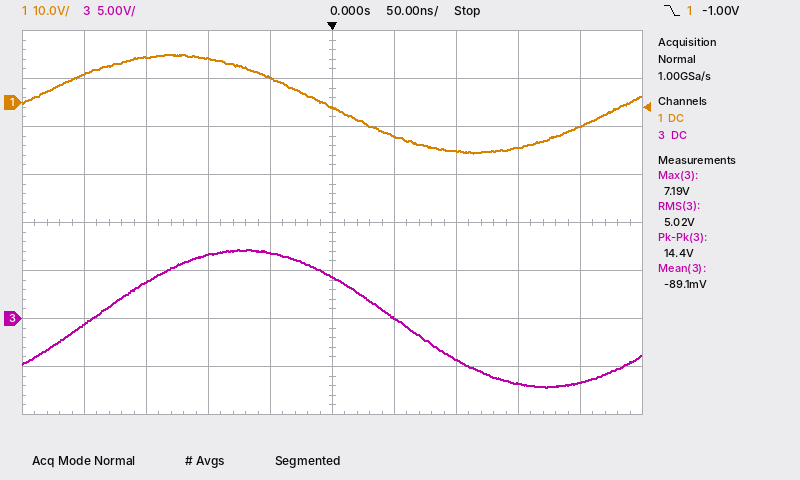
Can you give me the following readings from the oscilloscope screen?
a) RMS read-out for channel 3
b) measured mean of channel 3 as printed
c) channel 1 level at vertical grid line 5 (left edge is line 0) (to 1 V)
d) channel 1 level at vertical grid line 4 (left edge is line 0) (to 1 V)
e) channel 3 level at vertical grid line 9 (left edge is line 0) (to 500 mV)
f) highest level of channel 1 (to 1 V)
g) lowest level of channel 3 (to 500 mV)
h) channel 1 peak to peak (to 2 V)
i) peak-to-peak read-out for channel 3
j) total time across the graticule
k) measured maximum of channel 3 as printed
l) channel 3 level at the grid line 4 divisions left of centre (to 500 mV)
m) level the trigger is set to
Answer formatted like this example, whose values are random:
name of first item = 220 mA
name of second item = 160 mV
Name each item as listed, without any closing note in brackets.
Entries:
RMS read-out for channel 3 = 5.02 V
measured mean of channel 3 as printed = -89.1 mV
channel 1 level at vertical grid line 5 (left edge is line 0) = -1 V
channel 1 level at vertical grid line 4 (left edge is line 0) = 5 V
channel 3 level at vertical grid line 9 (left edge is line 0) = -6.5 V
highest level of channel 1 = 10 V
lowest level of channel 3 = -7.0 V
channel 1 peak to peak = 20 V
peak-to-peak read-out for channel 3 = 14.4 V
total time across the graticule = 500 ns
measured maximum of channel 3 as printed = 7.19 V
channel 3 level at the grid line 4 divisions left of centre = -500 mV
level the trigger is set to = -1.00 V
